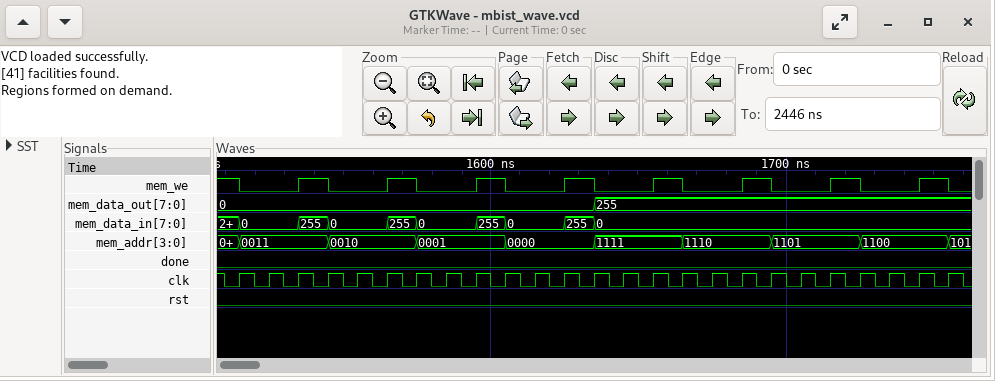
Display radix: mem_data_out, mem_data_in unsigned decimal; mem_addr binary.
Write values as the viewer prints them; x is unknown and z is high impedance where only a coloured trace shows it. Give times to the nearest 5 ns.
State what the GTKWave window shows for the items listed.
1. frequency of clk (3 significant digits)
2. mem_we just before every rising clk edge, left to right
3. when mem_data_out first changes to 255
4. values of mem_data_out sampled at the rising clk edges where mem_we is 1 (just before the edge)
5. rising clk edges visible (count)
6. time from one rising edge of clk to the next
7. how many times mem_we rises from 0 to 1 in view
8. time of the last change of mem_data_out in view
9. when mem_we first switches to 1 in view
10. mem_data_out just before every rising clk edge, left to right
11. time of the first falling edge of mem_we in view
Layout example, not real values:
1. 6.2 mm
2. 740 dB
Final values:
1. 100 MHz
2. 1 0 0 1 0 0 1 0 0 1 0 0 1 0 0 1 0 0 1 0 0 1 0 0 1
3. 1635 ns
4. 0, 0, 0, 0, 0, 255, 255, 255, 255
5. 25
6. 10 ns
7. 8
8. 1635 ns
9. 1535 ns
10. 0, 0, 0, 0, 0, 0, 0, 0, 0, 0, 0, 0, 0, 255, 255, 255, 255, 255, 255, 255, 255, 255, 255, 255, 255
11. 1515 ns
